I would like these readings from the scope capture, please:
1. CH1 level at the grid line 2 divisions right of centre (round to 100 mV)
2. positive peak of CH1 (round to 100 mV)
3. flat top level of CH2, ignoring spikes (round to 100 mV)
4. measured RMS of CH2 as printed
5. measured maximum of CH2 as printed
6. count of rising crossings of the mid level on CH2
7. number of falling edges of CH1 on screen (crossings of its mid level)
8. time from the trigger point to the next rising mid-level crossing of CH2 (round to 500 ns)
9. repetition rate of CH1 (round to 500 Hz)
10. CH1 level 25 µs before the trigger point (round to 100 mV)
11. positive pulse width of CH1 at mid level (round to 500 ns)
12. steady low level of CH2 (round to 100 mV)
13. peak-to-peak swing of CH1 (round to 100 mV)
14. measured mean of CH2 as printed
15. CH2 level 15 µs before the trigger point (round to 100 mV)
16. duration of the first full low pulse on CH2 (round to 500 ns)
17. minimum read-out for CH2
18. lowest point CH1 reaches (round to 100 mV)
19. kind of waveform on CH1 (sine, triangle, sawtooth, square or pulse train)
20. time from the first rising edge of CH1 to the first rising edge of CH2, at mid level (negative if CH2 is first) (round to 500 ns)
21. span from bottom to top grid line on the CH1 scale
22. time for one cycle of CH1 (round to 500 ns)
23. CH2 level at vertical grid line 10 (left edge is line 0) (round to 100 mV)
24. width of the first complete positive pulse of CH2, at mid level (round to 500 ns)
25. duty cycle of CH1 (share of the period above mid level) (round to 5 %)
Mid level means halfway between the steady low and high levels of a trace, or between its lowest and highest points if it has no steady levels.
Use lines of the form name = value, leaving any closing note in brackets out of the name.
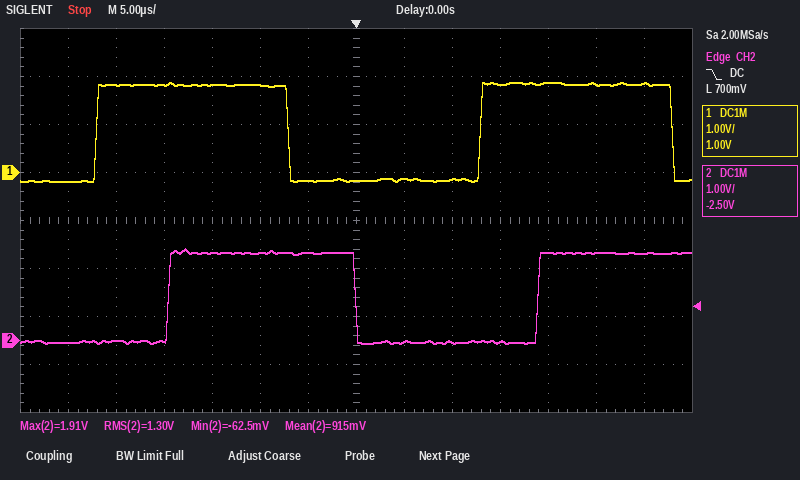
CH1 level at the grid line 2 divisions right of centre = -100 mV
positive peak of CH1 = 1.9 V
flat top level of CH2, ignoring spikes = 1.8 V
measured RMS of CH2 as printed = 1.30 V
measured maximum of CH2 as printed = 1.91 V
count of rising crossings of the mid level on CH2 = 2
number of falling edges of CH1 on screen = 2
time from the trigger point to the next rising mid-level crossing of CH2 = 19.0 µs
repetition rate of CH1 = 25.0 kHz
CH1 level 25 µs before the trigger point = 1.8 V
positive pulse width of CH1 at mid level = 20.0 µs
steady low level of CH2 = 0.0 V
peak-to-peak swing of CH1 = 2.1 V
measured mean of CH2 as printed = 915 mV
CH2 level 15 µs before the trigger point = 1.8 V
duration of the first full low pulse on CH2 = 19.0 µs
minimum read-out for CH2 = -62.5 mV
lowest point CH1 reaches = -200 mV
kind of waveform on CH1 = square
time from the first rising edge of CH1 to the first rising edge of CH2, at mid level (negative if CH2 is first) = +7.5 µs
span from bottom to top grid line on the CH1 scale = 8 V
time for one cycle of CH1 = 40.0 µs
CH2 level at vertical grid line 10 (left edge is line 0) = 0.0 V
width of the first complete positive pulse of CH2, at mid level = 19.5 µs
duty cycle of CH1 (share of the period above mid level) = 50 %
